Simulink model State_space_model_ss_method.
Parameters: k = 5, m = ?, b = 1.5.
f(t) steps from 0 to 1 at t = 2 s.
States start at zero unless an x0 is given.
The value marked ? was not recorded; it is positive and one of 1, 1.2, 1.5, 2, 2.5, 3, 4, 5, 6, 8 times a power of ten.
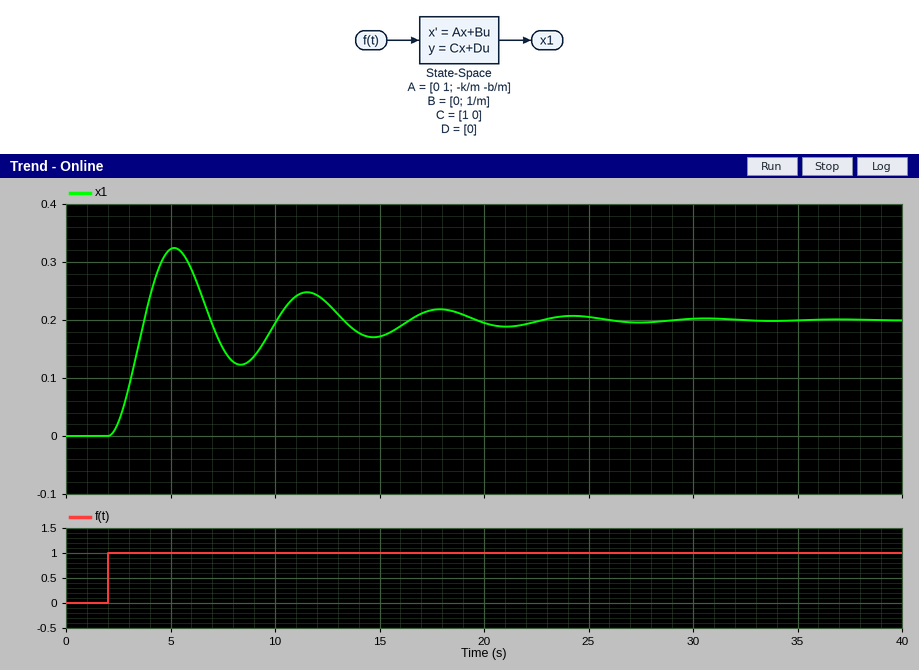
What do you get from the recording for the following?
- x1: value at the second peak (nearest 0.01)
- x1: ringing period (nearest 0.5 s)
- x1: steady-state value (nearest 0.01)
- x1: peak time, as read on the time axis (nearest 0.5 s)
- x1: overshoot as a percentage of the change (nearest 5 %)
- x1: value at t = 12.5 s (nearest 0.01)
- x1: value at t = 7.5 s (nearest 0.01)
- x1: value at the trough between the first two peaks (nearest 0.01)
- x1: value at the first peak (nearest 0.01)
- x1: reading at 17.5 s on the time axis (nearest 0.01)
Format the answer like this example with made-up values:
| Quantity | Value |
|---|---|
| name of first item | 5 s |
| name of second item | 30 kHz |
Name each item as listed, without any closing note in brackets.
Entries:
| Quantity | Value |
|---|---|
| x1: value at the second peak | 0.25 |
| x1: ringing period | 6.5 s |
| x1: steady-state value | 0.20 |
| x1: peak time, as read on the time axis | 5.0 s |
| x1: overshoot as a percentage of the change | 60 % |
| x1: value at t = 12.5 s | 0.23 |
| x1: value at t = 7.5 s | 0.15 |
| x1: value at the trough between the first two peaks | 0.12 |
| x1: value at the first peak | 0.32 |
| x1: reading at 17.5 s on the time axis | 0.22 |
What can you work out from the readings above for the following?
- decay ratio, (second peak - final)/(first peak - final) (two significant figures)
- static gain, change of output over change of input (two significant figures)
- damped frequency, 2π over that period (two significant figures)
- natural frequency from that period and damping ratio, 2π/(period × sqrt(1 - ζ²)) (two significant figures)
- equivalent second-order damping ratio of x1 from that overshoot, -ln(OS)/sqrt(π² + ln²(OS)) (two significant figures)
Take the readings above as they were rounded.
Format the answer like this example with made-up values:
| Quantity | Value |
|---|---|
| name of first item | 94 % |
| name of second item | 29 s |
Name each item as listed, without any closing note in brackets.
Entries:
| Quantity | Value |
|---|---|
| decay ratio, (second peak - final)/(first peak - final) | 0.42 |
| static gain, change of output over change of input | 0.20 |
| damped frequency, 2π over that period | 0.97 rad/s |
| natural frequency from that period and damping ratio, 2π/(period × sqrt(1 - ζ²)) | 0.98 rad/s |
| equivalent second-order damping ratio of x1 from that overshoot, -ln(OS)/sqrt(π² + ln²(OS)) | 0.16 |
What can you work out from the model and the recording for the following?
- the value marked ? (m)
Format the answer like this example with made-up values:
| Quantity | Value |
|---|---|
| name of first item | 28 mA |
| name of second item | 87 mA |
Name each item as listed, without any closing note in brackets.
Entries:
| Quantity | Value |
|---|---|
| the value marked ? | 5 |
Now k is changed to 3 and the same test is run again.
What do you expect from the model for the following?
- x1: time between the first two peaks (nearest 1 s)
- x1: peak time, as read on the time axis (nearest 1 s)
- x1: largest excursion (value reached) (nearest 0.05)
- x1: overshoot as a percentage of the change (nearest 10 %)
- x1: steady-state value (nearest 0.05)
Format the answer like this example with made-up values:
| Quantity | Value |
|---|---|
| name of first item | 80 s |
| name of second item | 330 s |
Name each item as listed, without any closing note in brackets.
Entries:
| Quantity | Value |
|---|---|
| x1: time between the first two peaks | 8 s |
| x1: peak time, as read on the time axis | 6 s |
| x1: largest excursion (value reached) | 0.50 |
| x1: overshoot as a percentage of the change | 50 % |
| x1: steady-state value | 0.35 |
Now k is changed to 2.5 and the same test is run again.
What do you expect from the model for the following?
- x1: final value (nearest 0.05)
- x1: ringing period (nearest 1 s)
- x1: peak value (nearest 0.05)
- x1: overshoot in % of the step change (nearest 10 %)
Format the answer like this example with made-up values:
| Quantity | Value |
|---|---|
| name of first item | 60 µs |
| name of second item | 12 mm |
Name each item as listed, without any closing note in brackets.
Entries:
| Quantity | Value |
|---|---|
| x1: final value | 0.40 |
| x1: ringing period | 9 s |
| x1: peak value | 0.60 |
| x1: overshoot in % of the step change | 50 % |
